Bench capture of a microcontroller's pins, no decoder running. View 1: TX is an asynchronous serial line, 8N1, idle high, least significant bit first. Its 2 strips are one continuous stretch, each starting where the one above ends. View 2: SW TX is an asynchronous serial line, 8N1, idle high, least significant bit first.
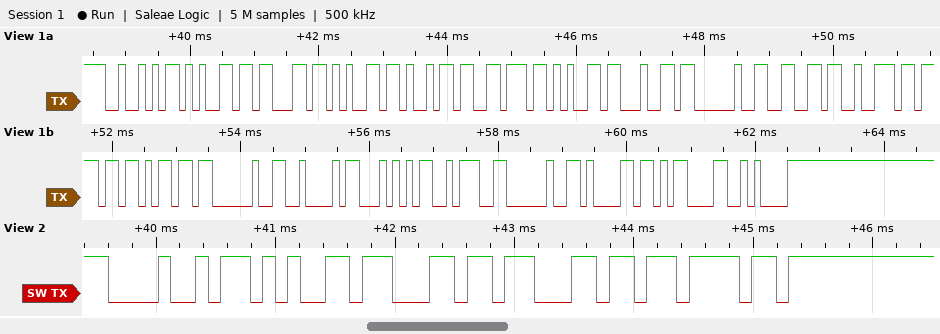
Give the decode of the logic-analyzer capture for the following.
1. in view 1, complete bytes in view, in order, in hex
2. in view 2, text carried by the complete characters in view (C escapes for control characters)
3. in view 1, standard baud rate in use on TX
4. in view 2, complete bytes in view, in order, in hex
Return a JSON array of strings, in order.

["52 65 63 65 69 76 65 64 20 66 72 6F 6D 20 42 54 3A 20 61 0D 0A", "\"Hello\"", "9600 baud", "0x48 0x65 0x6C 0x6C 0x6F"]
